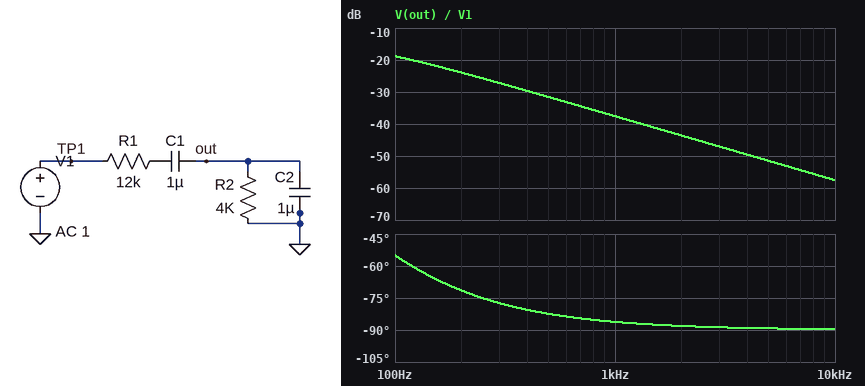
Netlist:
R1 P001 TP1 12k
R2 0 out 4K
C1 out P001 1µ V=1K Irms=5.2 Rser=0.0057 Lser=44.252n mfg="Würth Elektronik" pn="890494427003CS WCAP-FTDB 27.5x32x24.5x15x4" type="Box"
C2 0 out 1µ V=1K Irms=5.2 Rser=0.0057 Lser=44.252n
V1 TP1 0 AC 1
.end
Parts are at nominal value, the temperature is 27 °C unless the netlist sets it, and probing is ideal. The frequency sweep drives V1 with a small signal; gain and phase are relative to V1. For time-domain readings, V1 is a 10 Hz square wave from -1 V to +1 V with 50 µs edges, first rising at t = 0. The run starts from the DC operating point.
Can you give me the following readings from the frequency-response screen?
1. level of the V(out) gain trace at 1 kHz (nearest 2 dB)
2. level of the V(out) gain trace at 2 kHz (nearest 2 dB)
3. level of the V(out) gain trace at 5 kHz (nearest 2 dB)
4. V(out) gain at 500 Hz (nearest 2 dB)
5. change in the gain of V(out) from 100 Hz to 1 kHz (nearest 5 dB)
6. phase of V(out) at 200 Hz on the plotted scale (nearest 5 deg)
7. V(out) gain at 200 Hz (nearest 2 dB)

-38 dB
-44 dB
-52 dB
-32 dB
-20 dB
-70 deg
-24 dB
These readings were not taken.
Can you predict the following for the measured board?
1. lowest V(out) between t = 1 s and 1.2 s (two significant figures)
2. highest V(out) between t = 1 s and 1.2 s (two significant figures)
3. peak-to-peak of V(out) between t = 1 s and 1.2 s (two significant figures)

-310 mV
310 mV
610 mV
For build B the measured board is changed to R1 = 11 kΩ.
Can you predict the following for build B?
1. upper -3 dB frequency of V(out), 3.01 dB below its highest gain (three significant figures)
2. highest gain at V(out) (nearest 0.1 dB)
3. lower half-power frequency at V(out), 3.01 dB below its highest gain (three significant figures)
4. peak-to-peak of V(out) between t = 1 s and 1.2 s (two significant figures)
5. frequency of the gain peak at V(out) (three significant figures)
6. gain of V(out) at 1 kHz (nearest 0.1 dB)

76.3 Hz
-13.5 dB
7.55 Hz
650 mV
24.0 Hz
-36.8 dB
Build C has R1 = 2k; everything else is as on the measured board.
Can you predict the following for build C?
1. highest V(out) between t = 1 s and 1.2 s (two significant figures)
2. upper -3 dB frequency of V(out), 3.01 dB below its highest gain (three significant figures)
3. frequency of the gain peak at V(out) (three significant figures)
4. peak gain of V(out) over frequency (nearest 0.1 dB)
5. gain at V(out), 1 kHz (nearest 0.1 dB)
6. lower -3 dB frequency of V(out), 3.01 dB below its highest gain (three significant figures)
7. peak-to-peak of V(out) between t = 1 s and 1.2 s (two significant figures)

680 mV
214 Hz
56.3 Hz
-8.0 dB
-22.1 dB
14.8 Hz
1.4 V
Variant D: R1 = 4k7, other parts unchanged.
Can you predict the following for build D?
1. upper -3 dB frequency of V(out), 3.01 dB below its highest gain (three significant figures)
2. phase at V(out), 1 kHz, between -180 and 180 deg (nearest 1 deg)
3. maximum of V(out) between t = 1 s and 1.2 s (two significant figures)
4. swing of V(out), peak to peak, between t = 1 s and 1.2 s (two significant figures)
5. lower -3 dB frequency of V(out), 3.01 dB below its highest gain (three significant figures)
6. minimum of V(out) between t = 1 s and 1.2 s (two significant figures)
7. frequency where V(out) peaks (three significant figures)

119 Hz
-84 deg
510 mV
1.0 V
11.3 Hz
-510 mV
36.7 Hz
